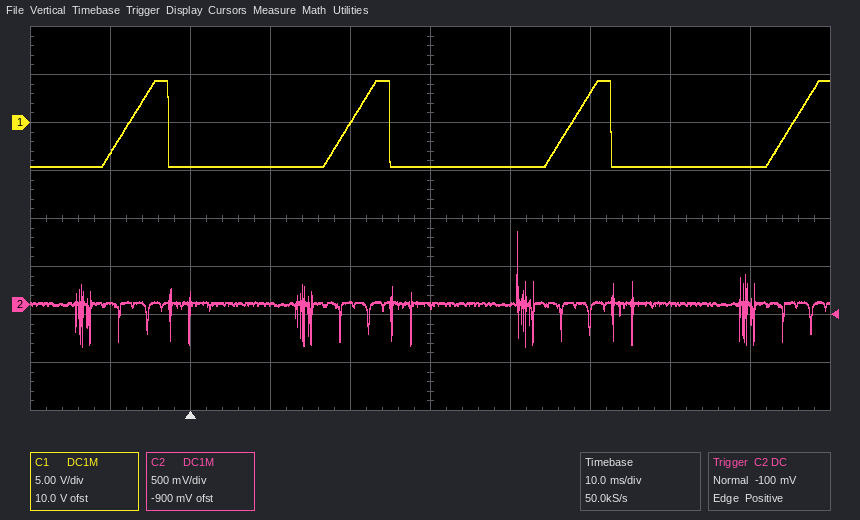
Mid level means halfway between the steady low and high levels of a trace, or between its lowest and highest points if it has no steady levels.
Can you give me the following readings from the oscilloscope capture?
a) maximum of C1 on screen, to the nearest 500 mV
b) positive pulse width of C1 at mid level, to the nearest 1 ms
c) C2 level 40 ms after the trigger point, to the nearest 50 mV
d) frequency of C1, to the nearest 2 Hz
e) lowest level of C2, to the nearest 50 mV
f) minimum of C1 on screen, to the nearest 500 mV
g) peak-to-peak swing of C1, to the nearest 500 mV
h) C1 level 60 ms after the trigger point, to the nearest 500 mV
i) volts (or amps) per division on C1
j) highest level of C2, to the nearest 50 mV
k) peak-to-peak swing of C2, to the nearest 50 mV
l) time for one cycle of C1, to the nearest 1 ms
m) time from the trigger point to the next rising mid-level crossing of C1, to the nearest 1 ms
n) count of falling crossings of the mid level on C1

4.5 V
5 ms
0 mV
36 Hz
-450 mV
-4.5 V
9.0 V
-4.5 V
5 V
750 mV
1.20 V
28 ms
20 ms
3
